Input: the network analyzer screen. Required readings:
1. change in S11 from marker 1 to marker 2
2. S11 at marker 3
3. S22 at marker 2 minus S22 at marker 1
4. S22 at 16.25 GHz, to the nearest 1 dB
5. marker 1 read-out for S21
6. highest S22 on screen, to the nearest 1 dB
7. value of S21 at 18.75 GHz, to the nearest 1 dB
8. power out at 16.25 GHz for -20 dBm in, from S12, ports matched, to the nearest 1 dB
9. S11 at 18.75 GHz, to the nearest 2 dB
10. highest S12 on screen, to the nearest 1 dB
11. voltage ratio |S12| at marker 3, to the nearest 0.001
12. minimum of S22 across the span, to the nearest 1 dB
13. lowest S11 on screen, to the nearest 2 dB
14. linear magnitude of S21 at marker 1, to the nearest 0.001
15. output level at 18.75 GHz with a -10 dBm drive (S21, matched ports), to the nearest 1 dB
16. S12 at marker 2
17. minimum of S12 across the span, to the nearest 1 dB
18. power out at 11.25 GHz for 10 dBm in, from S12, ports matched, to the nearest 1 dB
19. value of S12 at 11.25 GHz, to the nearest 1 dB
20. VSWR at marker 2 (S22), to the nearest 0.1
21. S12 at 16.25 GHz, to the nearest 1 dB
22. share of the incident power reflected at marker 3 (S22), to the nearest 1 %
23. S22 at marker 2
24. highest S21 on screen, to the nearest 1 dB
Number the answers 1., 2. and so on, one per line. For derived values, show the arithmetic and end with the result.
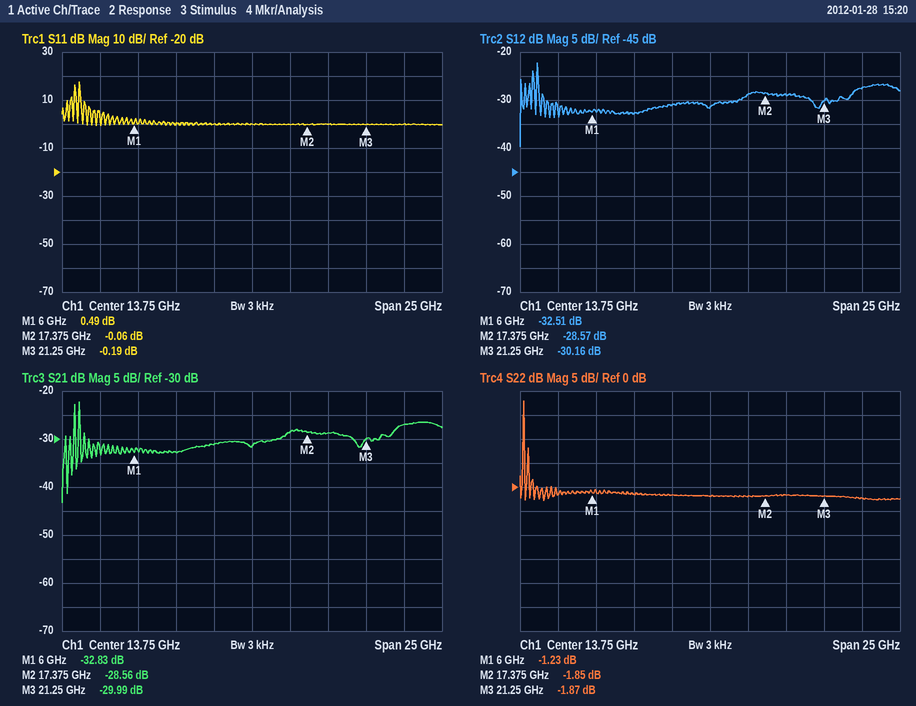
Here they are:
1. -0.06 − (0.49) = -0.55 dB
2. -0.19 dB
3. -1.85 − (-1.23) = -0.62 dB
4. -2 dB
5. -32.83 dB
6. 18 dB
7. -29 dB
8. -20 dBm + (-29 dB) = -49 dBm
9. 0 dB
10. -22 dB
11. 10^(-30.16/20) ≈ 0.031
12. -3 dB
13. 0 dB
14. 10^(-32.83/20) ≈ 0.023
15. -10 dBm + (-29 dB) = -39 dBm
16. -28.57 dB
17. -40 dB
18. 10 dBm + (-31 dB) = -21 dBm
19. -31 dB
20. (1 + 0.8082)/(1 − 0.8082) ≈ 9.4
21. -29 dB
22. 10^(-1.87/10) ≈ 65 %
23. -1.85 dB
24. -22 dB
